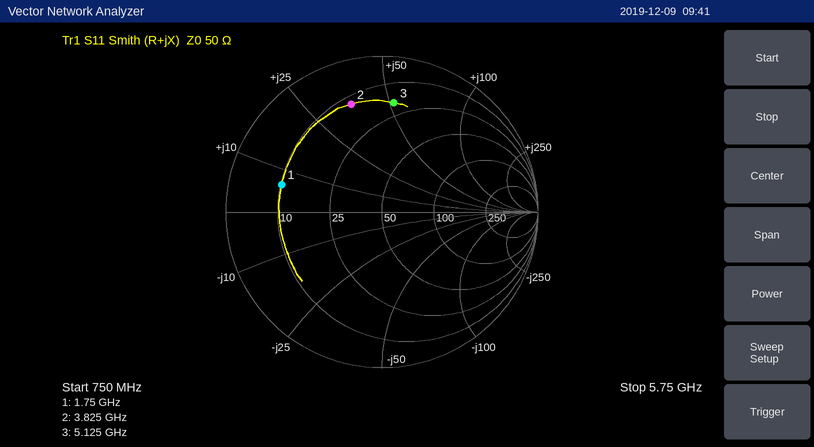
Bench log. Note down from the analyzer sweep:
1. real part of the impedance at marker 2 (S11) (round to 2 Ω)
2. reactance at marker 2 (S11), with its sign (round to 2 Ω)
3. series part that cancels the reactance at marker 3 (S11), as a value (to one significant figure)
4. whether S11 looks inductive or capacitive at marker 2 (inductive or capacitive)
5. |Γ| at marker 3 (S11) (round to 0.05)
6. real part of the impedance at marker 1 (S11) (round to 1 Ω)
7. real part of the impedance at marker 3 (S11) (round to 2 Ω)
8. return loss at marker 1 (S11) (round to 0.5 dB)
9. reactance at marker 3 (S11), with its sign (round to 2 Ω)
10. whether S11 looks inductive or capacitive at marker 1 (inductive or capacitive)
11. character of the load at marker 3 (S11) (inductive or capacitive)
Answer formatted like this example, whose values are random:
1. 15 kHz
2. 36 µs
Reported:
1. 12 Ω
2. +36 Ω
3. 600 fF
4. inductive
5. 0.70
6. 10 Ω
7. 18 Ω
8. 3.5 dB
9. +52 Ω
10. inductive
11. inductive
